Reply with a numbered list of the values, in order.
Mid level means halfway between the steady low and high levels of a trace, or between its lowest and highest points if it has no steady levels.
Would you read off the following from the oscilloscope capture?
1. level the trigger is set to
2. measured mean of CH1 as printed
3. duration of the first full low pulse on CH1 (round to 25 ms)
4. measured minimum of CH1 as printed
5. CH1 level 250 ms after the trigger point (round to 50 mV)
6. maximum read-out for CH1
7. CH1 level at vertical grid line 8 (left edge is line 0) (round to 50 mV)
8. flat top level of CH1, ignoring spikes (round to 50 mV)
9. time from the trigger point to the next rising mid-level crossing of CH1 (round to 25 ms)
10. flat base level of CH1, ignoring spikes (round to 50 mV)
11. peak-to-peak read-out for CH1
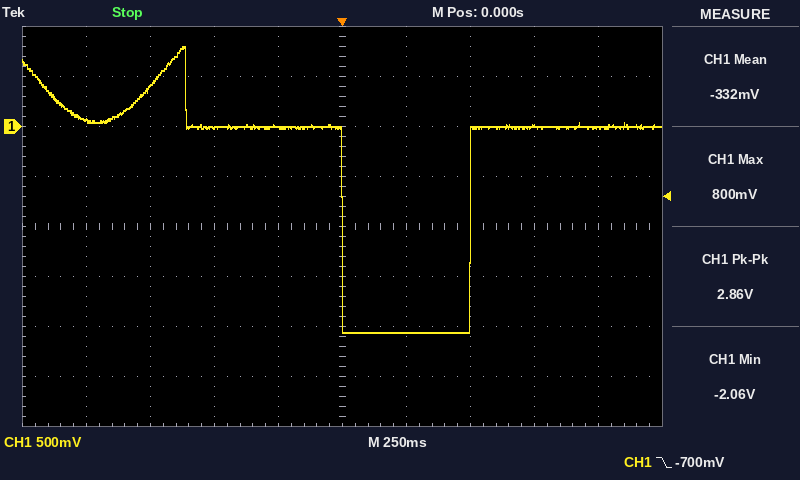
1. -700 mV
2. -332 mV
3. 500 ms
4. -2.06 V
5. -2.05 V
6. 800 mV
7. 0 mV
8. 0 mV
9. 500 ms
10. -2.05 V
11. 2.86 V
